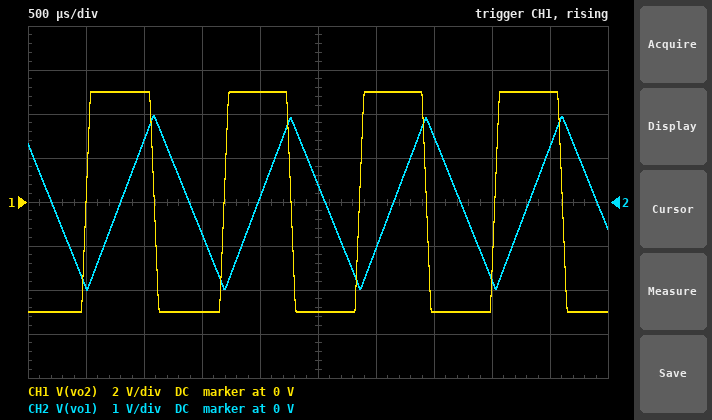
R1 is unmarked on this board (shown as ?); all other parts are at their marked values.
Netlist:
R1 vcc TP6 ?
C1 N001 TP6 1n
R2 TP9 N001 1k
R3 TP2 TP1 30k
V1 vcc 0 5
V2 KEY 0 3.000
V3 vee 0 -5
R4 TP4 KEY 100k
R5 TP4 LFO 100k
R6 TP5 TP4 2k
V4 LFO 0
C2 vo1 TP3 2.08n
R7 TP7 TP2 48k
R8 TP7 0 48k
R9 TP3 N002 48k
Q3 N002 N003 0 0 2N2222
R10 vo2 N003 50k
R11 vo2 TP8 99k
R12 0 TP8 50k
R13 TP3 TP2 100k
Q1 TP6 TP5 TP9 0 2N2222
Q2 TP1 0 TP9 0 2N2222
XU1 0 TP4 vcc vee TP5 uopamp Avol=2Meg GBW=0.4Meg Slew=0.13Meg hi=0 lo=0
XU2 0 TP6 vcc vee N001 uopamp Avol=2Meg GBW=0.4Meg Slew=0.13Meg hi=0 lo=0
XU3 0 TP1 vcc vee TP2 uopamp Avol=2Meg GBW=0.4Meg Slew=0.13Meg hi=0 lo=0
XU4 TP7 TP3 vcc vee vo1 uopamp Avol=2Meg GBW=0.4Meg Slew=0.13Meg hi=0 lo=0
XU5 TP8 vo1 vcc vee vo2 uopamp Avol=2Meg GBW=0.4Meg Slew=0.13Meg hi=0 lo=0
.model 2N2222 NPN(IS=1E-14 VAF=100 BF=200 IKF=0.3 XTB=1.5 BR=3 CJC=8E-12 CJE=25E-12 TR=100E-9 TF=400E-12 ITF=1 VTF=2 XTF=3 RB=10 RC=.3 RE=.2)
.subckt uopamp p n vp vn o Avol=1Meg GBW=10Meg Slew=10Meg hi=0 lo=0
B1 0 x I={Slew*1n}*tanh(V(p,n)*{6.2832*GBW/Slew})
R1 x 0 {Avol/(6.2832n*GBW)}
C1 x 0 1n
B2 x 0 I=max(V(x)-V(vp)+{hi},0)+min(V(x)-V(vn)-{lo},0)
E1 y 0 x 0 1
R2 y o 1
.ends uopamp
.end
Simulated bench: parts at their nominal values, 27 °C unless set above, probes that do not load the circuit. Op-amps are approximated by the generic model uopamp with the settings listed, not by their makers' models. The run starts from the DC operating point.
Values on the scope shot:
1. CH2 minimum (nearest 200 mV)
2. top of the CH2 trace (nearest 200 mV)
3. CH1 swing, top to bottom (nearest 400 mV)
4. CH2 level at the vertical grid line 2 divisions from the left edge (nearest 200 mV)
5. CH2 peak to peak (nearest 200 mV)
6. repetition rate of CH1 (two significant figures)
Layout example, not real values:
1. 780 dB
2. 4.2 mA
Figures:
1. -2.0 V
2. 2.0 V
3. 10.0 V
4. 1.4 V
5. 4.0 V
6. 850 Hz
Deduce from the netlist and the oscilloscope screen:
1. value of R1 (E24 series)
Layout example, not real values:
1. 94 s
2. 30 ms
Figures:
1. 560 kΩ
